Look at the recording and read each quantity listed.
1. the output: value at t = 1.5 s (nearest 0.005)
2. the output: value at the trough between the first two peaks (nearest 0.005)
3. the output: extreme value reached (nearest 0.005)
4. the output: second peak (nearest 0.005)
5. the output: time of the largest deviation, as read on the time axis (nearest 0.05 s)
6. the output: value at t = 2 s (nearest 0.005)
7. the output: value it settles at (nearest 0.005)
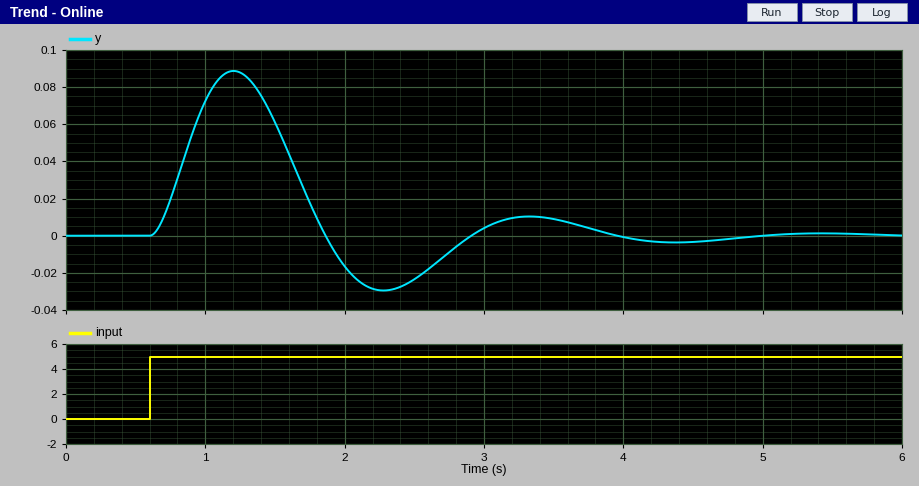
0.060
-0.030
0.090
0.010
1.20 s
-0.015
0.000
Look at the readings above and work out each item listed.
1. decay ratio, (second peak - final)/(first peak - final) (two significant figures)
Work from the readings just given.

0.11
